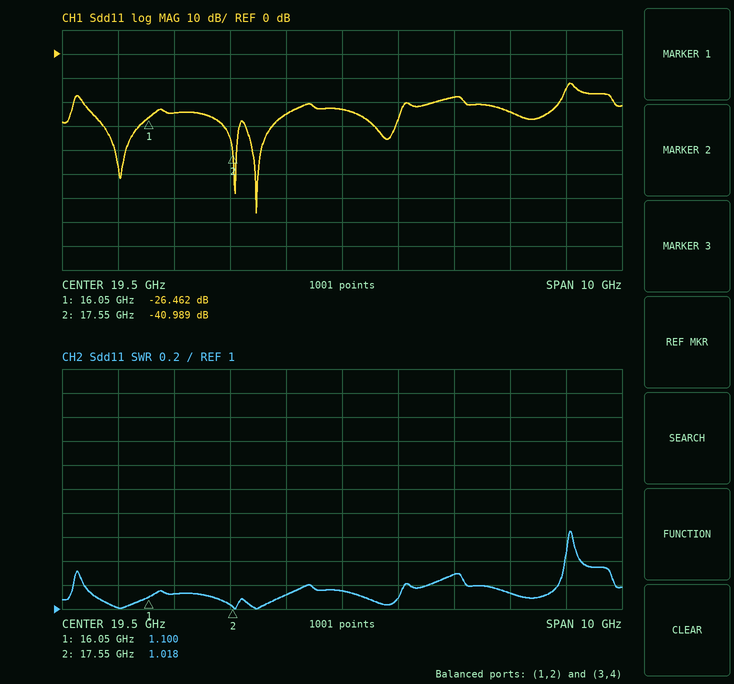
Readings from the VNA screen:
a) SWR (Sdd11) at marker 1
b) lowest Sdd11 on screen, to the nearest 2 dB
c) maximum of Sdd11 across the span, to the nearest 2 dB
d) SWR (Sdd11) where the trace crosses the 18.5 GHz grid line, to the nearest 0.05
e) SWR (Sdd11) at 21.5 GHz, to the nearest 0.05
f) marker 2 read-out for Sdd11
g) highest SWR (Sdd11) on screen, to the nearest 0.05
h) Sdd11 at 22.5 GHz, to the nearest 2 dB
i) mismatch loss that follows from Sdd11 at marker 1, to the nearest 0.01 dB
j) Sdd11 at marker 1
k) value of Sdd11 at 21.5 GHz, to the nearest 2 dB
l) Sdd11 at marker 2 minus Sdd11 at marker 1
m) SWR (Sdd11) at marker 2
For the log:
1.100
-66 dB
-12 dB
1.10
1.30
-40.989 dB
1.65
-24 dB
0.01 dB
-26.462 dB
-18 dB
-14.527 dB
1.018
